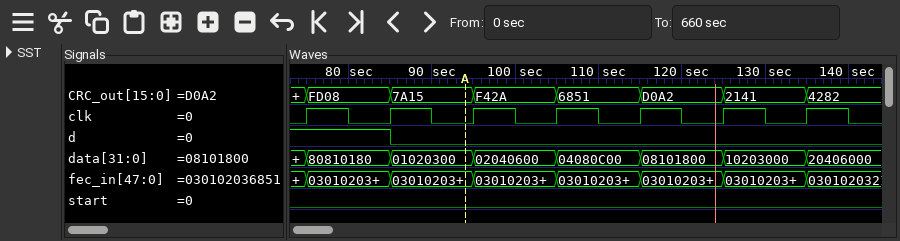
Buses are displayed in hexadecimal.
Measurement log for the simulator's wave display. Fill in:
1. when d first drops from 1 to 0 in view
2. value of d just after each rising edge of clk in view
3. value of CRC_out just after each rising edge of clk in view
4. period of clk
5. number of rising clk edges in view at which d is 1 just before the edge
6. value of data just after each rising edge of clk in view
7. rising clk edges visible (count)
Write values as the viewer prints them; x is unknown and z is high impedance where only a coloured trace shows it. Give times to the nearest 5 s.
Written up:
85 s
1 0 0 0 0 0 0
FD08, 7A15, F42A, 6851, D0A2, 2141, 4282
10 s
2
80810180, 01020300, 02040600, 04080C00, 08101800, 10203000, 20406000
7
